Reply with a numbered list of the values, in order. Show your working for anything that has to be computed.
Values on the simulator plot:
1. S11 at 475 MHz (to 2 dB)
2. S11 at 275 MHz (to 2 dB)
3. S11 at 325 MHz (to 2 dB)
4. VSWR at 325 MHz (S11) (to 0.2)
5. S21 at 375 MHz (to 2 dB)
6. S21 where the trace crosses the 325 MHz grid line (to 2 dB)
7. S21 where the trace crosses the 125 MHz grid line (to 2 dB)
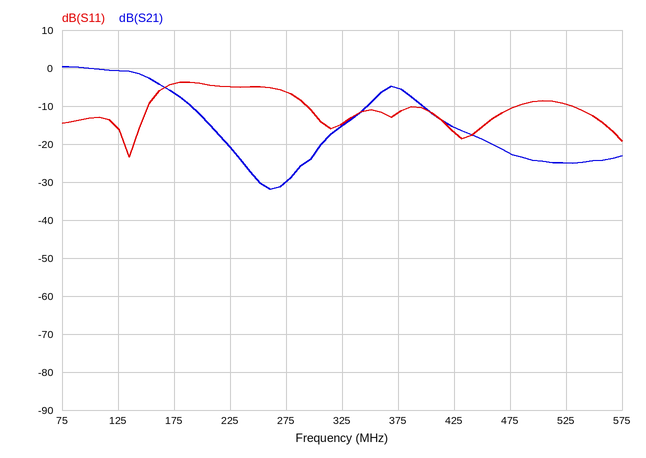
1. -10 dB
2. -6 dB
3. -14 dB
4. |Γ| = 10^(-14/20) = 0.1995; VSWR = (1 + 0.1995)/(1 − 0.1995) ≈ 1.50, so 1.4 to the nearest 0.2
5. -6 dB
6. -16 dB
7. 0 dB
